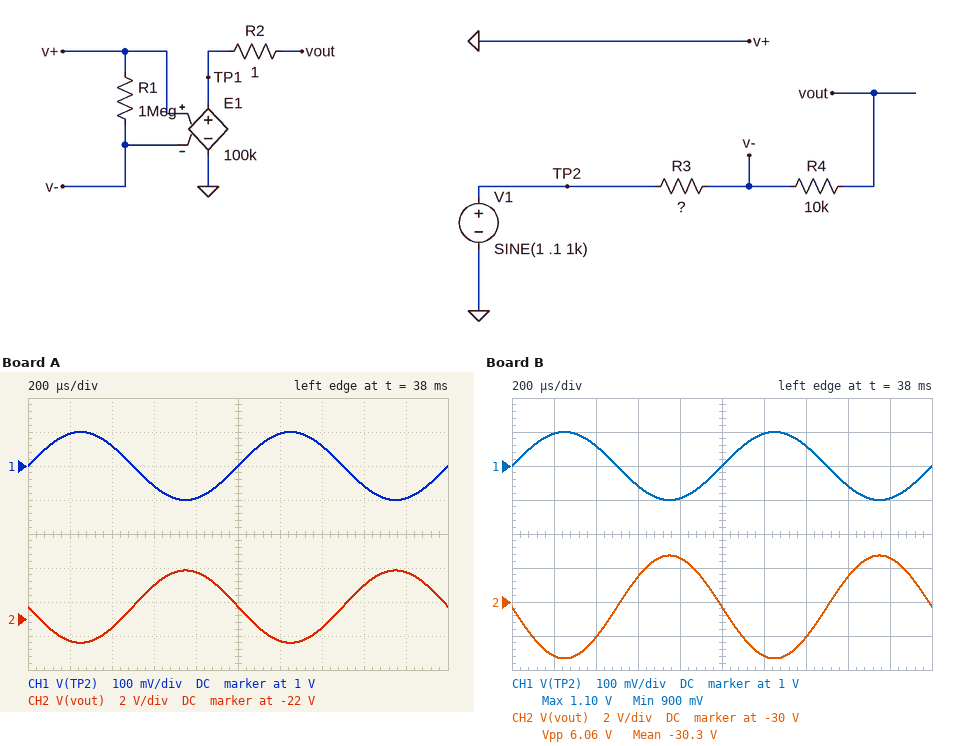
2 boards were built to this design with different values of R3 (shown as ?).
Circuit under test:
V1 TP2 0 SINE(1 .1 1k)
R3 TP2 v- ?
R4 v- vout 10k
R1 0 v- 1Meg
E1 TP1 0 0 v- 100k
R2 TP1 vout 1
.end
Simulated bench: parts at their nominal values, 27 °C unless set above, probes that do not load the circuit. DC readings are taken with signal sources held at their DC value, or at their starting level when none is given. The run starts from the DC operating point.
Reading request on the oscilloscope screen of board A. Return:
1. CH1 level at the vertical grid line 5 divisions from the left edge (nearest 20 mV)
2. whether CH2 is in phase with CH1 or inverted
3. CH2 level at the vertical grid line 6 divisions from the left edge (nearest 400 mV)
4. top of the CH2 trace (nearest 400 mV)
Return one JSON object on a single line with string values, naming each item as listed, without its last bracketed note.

{"CH1 level at the vertical grid line 5 divisions from the left edge": "1.00 V", "whether CH2 is in phase with CH1 or inverted": "inverted", "CH2 level at the vertical grid line 6 divisions from the left edge": "-23.2 V", "top of the CH2 trace": "-19.2 V"}
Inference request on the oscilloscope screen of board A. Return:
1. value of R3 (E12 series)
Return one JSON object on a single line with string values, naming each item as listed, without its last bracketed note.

{"value of R3": "470 Ω"}
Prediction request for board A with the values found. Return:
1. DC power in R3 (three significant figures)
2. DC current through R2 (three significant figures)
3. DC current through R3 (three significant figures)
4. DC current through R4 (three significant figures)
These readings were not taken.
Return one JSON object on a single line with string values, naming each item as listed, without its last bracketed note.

{"DC power in R3": "2.13 mW", "DC current through R2": "2.13 mA", "DC current through R3": "2.13 mA", "DC current through R4": "2.13 mA"}
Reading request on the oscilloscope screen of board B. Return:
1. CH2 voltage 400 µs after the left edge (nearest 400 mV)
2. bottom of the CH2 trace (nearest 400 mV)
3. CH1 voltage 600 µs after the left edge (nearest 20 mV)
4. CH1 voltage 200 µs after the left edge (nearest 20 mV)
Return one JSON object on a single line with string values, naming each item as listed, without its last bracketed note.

{"CH2 voltage 400 µs after the left edge": "-32.0 V", "bottom of the CH2 trace": "-33.2 V", "CH1 voltage 600 µs after the left edge": "940 mV", "CH1 voltage 200 µs after the left edge": "1.10 V"}
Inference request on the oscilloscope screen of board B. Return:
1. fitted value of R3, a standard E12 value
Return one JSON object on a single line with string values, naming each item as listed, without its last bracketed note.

{"fitted value of R3, a standard E12 value": "330 Ω"}
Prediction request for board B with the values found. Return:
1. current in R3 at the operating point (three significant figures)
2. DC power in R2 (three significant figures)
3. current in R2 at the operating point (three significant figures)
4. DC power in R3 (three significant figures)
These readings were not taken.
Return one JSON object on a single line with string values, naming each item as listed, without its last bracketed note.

{"current in R3 at the operating point": "3.03 mA", "DC power in R2": "9.18 µW", "current in R2 at the operating point": "3.03 mA", "DC power in R3": "3.03 mW"}
